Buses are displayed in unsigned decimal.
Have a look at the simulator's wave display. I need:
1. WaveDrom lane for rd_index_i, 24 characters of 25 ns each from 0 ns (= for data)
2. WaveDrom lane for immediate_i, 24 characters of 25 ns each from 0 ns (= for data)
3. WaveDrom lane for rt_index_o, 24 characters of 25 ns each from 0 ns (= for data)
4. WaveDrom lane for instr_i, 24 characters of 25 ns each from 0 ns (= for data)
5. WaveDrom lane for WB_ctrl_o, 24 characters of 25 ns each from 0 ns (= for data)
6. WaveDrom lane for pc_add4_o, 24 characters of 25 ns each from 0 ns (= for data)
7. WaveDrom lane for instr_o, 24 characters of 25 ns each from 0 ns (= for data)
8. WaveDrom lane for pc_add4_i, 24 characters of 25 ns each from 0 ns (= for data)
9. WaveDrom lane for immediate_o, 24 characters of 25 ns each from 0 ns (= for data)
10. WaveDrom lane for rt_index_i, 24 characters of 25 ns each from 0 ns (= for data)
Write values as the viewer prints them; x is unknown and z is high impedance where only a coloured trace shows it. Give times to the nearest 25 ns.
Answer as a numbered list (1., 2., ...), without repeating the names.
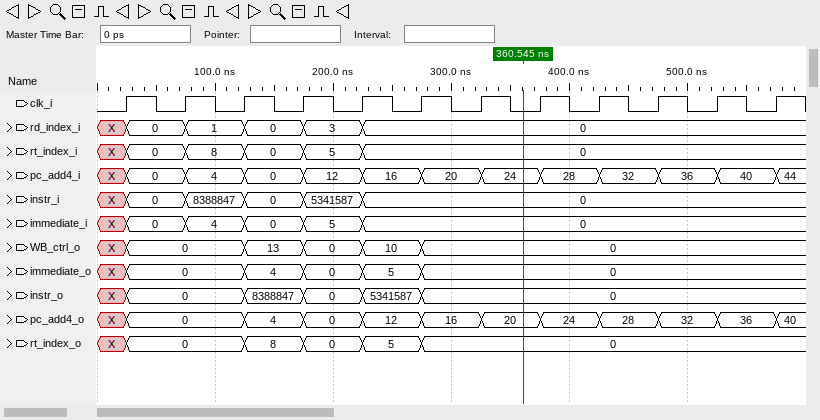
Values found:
1. {name: 'rd_index_i', wave: 'x=.=.=.=.=..............', data: '0 1 0 3 0'}
2. {name: 'immediate_i', wave: 'x=.=.=.=.=..............', data: '0 4 0 5 0'}
3. {name: 'rt_index_o', wave: 'x=...=.=.=.=............', data: '0 8 0 5 0'}
4. {name: 'instr_i', wave: 'x=.=.=.=.=..............', data: '0 8388847 0 5341587 0'}
5. {name: 'WB_ctrl_o', wave: 'x=...=.=.=.=............', data: '0 13 0 10 0'}
6. {name: 'pc_add4_o', wave: 'x=...=.=.=.=.=.=.=.=.=.=', data: '0 4 0 12 16 20 24 28 32 36 40'}
7. {name: 'instr_o', wave: 'x=...=.=.=.=............', data: '0 8388847 0 5341587 0'}
8. {name: 'pc_add4_i', wave: 'x=.=.=.=.=.=.=.=.=.=.=.=', data: '0 4 0 12 16 20 24 28 32 36 40 44'}
9. {name: 'immediate_o', wave: 'x=...=.=.=.=............', data: '0 4 0 5 0'}
10. {name: 'rt_index_i', wave: 'x=.=.=.=.=..............', data: '0 8 0 5 0'}
